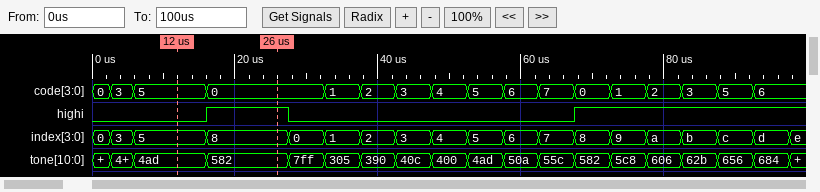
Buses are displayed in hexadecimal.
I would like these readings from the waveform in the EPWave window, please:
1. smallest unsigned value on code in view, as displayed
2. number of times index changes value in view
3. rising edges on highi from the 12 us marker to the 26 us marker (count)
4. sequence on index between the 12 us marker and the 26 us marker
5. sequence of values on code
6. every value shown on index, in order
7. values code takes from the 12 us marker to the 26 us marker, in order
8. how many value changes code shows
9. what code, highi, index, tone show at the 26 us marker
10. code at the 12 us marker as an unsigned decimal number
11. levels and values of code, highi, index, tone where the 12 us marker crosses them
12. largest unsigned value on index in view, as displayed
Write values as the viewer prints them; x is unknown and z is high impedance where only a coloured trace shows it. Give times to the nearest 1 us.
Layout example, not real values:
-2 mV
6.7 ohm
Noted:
0
18
1
5, 8
0, 3, 5, 0, 1, 2, 3, 4, 5, 6, 7, 0, 1, 2, 3, 5, 6
0, 3, 5, 8, 0, 1, 2, 3, 4, 5, 6, 7, 8, 9, a, b, c, d, e
5, 0
16
code=0, highi=1, index=8, tone=582
5
code=5, highi=0, index=5, tone=4ad
e
